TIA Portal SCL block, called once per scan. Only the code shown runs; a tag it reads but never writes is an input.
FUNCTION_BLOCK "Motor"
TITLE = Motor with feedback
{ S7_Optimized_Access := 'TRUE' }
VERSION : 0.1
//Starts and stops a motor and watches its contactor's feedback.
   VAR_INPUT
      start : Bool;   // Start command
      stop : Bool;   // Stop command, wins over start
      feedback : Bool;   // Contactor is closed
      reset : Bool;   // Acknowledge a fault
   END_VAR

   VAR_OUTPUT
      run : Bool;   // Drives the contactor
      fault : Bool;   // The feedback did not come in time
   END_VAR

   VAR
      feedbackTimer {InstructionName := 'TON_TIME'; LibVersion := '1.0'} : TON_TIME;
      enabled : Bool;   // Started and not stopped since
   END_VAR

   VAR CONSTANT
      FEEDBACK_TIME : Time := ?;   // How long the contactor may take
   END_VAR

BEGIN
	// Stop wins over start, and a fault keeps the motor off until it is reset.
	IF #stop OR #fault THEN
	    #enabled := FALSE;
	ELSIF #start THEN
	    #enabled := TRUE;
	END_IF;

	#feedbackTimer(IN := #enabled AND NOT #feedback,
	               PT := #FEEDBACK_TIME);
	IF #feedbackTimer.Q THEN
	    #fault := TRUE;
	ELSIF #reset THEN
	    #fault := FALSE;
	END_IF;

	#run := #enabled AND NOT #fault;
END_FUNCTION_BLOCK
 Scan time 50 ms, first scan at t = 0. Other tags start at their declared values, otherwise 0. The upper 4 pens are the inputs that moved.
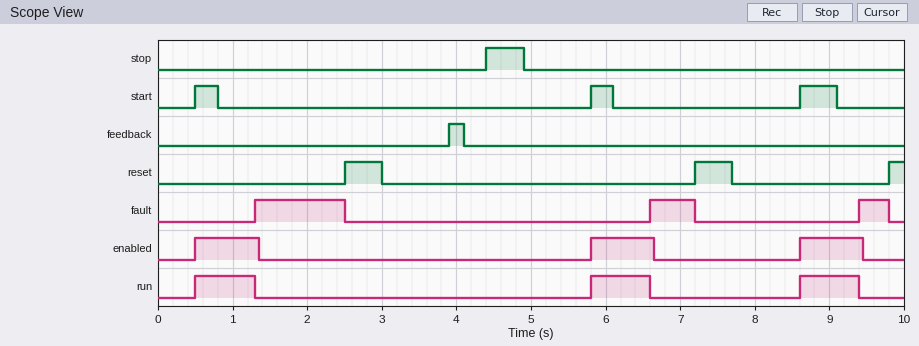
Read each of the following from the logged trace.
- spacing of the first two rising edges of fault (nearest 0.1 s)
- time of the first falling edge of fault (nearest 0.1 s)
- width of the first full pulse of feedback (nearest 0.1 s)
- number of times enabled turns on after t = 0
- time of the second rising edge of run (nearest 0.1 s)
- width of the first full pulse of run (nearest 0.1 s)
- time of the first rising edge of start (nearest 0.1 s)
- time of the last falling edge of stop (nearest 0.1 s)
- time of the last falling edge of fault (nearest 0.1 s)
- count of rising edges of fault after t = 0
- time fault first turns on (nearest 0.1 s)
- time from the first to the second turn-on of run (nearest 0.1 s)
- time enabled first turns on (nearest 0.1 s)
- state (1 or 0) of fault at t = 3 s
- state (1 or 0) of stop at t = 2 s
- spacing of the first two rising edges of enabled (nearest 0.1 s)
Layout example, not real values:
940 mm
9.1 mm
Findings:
5.3 s
2.5 s
0.2 s
3
5.8 s
0.8 s
0.5 s
4.9 s
9.8 s
3
1.3 s
5.3 s
0.5 s
0
0
5.3 s
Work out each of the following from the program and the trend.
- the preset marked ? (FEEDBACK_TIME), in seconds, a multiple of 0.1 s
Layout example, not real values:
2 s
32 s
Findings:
0.8 s
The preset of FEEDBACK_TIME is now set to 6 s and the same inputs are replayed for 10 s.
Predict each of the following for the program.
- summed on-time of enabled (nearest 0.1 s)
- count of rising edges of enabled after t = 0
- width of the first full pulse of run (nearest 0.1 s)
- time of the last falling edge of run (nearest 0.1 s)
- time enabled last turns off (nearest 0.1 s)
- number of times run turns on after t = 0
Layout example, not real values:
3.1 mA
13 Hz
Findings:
8.1 s
2
3.9 s
4.4 s
4.4 s
2
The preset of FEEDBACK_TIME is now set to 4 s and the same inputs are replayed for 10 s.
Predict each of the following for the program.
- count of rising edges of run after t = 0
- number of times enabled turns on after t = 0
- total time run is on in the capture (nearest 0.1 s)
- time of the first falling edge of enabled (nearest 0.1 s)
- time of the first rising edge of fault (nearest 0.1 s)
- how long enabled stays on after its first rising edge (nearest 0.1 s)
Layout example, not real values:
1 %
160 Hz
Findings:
2
2
7.9 s
4.4 s
9.8 s
3.9 s
